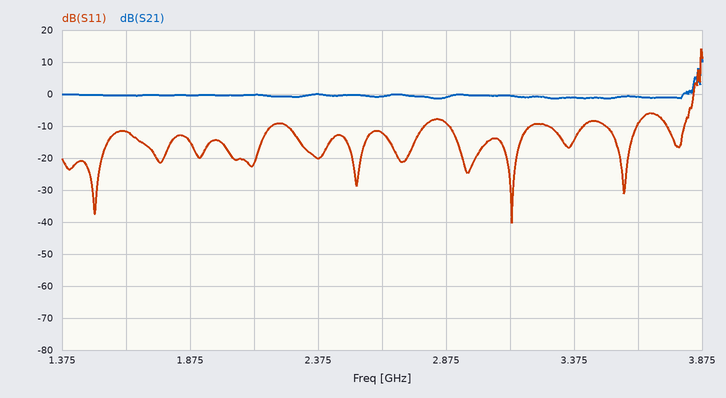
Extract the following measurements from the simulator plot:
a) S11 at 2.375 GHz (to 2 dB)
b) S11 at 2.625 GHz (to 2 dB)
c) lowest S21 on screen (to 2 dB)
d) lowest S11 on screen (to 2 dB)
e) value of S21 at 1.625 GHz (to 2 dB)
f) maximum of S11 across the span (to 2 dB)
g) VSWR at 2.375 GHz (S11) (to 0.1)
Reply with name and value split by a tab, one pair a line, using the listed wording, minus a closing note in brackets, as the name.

S11 at 2.375 GHz	-20 dB
S11 at 2.625 GHz	-12 dB
lowest S21 on screen	-2 dB
lowest S11 on screen	-40 dB
value of S21 at 1.625 GHz	0 dB
maximum of S11 across the span	14 dB
VSWR at 2.375 GHz (S11)	1.2
